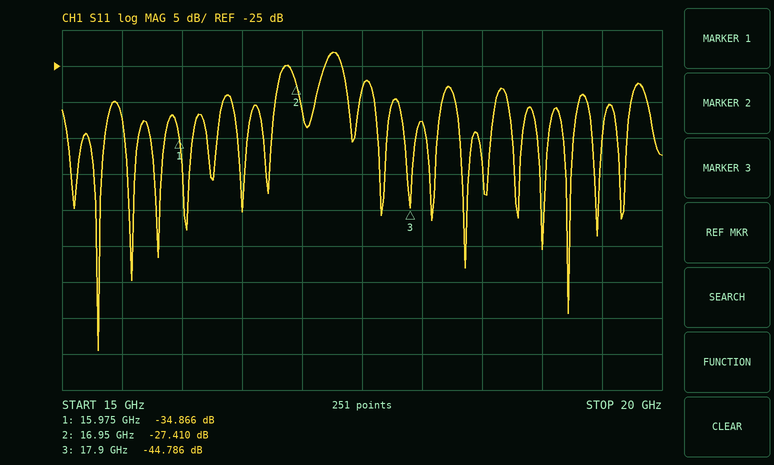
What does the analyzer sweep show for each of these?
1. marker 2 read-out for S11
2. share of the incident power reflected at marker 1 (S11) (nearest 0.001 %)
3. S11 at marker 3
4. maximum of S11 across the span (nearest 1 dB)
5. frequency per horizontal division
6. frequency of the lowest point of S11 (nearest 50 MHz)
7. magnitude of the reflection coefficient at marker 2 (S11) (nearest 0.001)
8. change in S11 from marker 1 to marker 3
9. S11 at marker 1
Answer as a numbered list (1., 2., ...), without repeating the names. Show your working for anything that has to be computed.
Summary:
1. -27.410 dB
2. 10^(-34.866/10) ≈ 0.033 %
3. -44.786 dB
4. -23 dB
5. 500 MHz
6. 15.30 GHz
7. 10^(-27.41/20) ≈ 0.043
8. -44.786 − (-34.866) = -9.920 dB
9. -34.866 dB
